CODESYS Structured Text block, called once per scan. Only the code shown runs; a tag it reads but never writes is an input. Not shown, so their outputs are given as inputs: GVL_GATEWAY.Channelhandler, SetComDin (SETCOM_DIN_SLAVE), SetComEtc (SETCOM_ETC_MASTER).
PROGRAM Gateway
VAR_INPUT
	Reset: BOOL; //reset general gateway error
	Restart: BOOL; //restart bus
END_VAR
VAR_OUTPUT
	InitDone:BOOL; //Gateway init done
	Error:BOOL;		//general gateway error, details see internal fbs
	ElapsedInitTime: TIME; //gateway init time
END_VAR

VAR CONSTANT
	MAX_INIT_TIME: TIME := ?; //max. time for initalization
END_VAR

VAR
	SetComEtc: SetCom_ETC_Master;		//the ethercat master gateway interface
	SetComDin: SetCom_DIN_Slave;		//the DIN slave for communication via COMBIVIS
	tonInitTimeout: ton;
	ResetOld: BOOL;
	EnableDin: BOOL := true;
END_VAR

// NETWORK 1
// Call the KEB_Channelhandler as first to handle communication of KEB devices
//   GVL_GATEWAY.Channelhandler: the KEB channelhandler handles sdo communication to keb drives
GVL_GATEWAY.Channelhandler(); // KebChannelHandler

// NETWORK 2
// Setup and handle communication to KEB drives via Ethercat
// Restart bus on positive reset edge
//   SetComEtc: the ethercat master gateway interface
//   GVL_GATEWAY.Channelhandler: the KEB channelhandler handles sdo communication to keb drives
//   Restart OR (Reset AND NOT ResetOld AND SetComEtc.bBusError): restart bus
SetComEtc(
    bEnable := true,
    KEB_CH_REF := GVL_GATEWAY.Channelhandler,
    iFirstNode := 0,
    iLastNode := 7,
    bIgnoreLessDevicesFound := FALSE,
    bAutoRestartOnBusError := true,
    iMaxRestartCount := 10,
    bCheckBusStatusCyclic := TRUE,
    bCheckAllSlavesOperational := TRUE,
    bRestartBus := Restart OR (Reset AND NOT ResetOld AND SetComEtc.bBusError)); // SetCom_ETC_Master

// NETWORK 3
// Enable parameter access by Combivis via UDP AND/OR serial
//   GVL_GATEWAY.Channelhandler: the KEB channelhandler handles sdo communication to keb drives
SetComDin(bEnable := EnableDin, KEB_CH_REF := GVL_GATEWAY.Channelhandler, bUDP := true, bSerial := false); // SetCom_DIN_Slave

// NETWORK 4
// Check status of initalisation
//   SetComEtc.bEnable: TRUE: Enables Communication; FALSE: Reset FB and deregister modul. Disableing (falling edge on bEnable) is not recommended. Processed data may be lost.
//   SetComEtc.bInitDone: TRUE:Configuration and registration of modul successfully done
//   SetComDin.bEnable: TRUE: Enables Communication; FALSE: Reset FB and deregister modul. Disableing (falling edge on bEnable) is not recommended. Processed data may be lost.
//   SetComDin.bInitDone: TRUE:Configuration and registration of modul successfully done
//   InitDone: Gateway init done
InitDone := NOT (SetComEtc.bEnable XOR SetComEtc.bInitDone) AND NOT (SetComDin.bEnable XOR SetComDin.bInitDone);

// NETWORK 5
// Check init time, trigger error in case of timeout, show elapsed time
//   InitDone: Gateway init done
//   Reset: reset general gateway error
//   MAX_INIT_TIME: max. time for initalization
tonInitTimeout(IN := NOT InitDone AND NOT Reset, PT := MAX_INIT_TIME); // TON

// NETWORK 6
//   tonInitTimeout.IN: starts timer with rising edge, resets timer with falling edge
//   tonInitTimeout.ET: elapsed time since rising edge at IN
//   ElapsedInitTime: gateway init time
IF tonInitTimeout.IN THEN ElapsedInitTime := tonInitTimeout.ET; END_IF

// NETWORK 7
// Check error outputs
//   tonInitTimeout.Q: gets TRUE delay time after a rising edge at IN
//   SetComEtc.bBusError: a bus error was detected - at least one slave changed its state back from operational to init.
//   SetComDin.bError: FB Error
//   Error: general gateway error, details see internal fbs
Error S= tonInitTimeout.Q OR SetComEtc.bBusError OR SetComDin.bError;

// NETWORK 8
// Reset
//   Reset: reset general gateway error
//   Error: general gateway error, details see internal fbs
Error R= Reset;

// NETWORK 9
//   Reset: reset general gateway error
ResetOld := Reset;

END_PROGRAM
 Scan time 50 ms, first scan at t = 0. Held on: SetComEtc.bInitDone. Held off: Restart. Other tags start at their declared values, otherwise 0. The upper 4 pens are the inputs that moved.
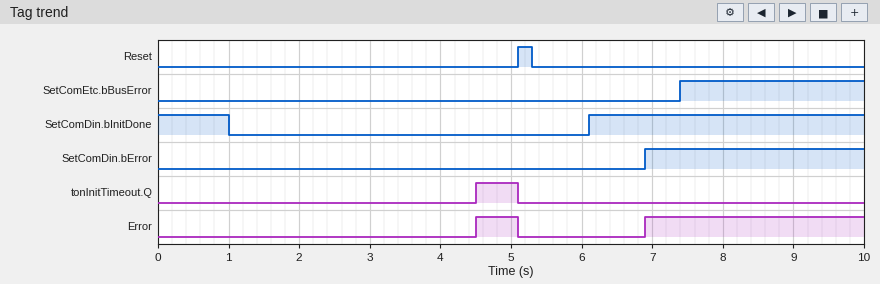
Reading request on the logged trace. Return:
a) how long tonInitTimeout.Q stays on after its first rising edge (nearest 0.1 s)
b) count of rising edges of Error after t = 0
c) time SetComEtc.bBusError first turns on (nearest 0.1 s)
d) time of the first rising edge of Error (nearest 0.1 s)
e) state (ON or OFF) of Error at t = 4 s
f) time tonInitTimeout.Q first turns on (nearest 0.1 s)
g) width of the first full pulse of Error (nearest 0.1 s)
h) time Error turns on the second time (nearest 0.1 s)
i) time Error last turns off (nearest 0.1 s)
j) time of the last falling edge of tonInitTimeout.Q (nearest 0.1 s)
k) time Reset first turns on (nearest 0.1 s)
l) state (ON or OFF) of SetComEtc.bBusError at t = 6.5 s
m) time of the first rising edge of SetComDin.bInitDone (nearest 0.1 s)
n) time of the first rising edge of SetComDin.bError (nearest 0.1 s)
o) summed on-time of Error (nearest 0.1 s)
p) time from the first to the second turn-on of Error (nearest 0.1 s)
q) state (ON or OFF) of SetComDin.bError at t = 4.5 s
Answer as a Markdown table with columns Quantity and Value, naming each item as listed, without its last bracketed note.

| Quantity | Value |
|---|---|
| how long tonInitTimeout.Q stays on after its first rising edge | 0.6 s |
| count of rising edges of Error after t = 0 | 2 |
| time SetComEtc.bBusError first turns on | 7.4 s |
| time of the first rising edge of Error | 4.5 s |
| state (ON or OFF) of Error at t = 4 s | OFF |
| time tonInitTimeout.Q first turns on | 4.5 s |
| width of the first full pulse of Error | 0.6 s |
| time Error turns on the second time | 6.9 s |
| time Error last turns off | 5.1 s |
| time of the last falling edge of tonInitTimeout.Q | 5.1 s |
| time Reset first turns on | 5.1 s |
| state (ON or OFF) of SetComEtc.bBusError at t = 6.5 s | OFF |
| time of the first rising edge of SetComDin.bInitDone | 6.1 s |
| time of the first rising edge of SetComDin.bError | 6.9 s |
| summed on-time of Error | 3.7 s |
| time from the first to the second turn-on of Error | 2.4 s |
| state (ON or OFF) of SetComDin.bError at t = 4.5 s | OFF |
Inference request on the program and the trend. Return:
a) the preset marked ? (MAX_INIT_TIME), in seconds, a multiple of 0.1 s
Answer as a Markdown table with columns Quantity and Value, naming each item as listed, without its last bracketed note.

| Quantity | Value |
|---|---|
| the preset marked ? (MAX_INIT_TIME), in seconds, a multiple of 0.1 s | 3.5 s |
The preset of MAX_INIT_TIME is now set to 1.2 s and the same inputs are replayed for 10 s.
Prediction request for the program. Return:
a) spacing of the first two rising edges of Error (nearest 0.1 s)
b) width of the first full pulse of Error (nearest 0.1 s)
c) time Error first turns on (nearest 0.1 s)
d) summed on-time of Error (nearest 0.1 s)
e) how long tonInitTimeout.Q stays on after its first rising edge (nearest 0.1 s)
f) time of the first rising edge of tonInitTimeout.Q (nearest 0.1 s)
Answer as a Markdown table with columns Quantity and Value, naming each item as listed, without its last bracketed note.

| Quantity | Value |
|---|---|
| spacing of the first two rising edges of Error | 4.7 s |
| width of the first full pulse of Error | 2.9 s |
| time Error first turns on | 2.2 s |
| summed on-time of Error | 6.0 s |
| how long tonInitTimeout.Q stays on after its first rising edge | 2.9 s |
| time of the first rising edge of tonInitTimeout.Q | 2.2 s |
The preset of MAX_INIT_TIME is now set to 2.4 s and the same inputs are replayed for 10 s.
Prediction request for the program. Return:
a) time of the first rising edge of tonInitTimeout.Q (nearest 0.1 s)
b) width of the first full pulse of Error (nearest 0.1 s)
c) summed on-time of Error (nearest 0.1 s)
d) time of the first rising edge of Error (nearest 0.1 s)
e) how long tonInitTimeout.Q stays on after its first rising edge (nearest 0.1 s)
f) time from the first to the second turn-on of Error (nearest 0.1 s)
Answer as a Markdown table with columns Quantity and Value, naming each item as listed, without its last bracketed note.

| Quantity | Value |
|---|---|
| time of the first rising edge of tonInitTimeout.Q | 3.4 s |
| width of the first full pulse of Error | 1.7 s |
| summed on-time of Error | 4.8 s |
| time of the first rising edge of Error | 3.4 s |
| how long tonInitTimeout.Q stays on after its first rising edge | 1.7 s |
| time from the first to the second turn-on of Error | 3.5 s |
